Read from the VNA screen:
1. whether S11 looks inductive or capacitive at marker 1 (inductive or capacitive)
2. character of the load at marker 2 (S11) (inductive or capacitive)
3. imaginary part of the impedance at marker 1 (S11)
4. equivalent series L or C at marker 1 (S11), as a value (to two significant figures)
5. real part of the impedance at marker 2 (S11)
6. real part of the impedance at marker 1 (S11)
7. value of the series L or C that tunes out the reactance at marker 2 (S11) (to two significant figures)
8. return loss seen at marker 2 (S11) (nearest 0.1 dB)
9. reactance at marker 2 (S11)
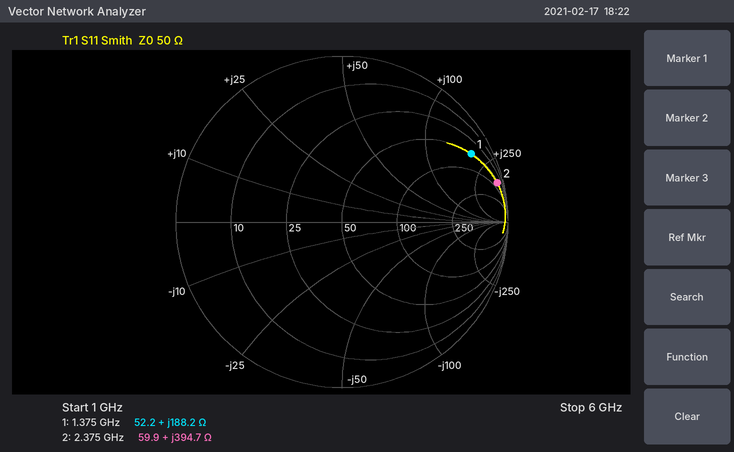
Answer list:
inductive
inductive
+188.2 Ω
22 nH
59.9 Ω
52.2 Ω
170 fF
0.3 dB
+394.7 Ω
